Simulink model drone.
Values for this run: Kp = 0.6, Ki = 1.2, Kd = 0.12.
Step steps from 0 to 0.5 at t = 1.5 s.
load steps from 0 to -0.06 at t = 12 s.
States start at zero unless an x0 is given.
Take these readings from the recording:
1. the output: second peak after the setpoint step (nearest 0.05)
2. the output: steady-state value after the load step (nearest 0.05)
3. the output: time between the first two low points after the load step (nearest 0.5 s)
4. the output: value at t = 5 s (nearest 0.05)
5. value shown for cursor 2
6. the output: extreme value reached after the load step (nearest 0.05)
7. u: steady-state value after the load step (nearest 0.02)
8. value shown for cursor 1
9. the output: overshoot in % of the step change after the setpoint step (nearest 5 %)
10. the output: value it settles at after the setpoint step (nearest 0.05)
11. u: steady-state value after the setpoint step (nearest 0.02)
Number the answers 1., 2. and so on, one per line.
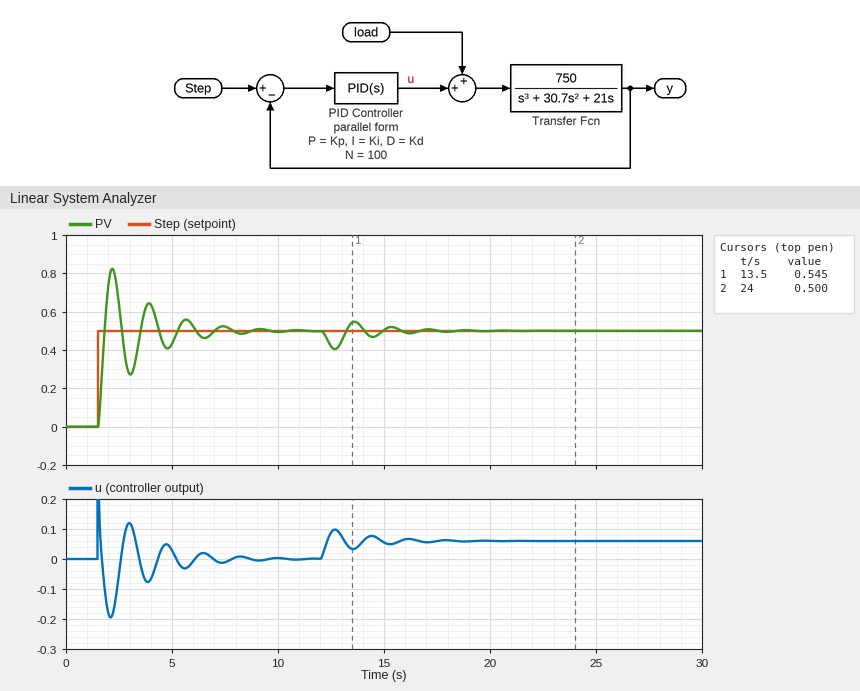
1. 0.65
2. 0.50
3. 2.0 s
4. 0.45
5. 0.500
6. 0.40
7. 0.06
8. 0.545
9. 65 %
10. 0.50
11. 0.00
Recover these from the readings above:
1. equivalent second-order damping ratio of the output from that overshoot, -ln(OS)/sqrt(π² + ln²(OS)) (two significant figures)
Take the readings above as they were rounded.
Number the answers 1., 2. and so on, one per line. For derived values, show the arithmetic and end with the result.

1. ln(0.65) = -0.431; 0.431 / sqrt(9.870 + 0.186) = 0.14
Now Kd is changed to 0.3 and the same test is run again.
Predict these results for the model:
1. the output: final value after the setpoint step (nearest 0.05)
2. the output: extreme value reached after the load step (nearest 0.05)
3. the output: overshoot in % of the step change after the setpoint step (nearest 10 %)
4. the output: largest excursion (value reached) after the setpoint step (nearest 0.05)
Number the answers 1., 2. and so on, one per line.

1. 0.50
2. 0.45
3. 20 %
4. 0.60
